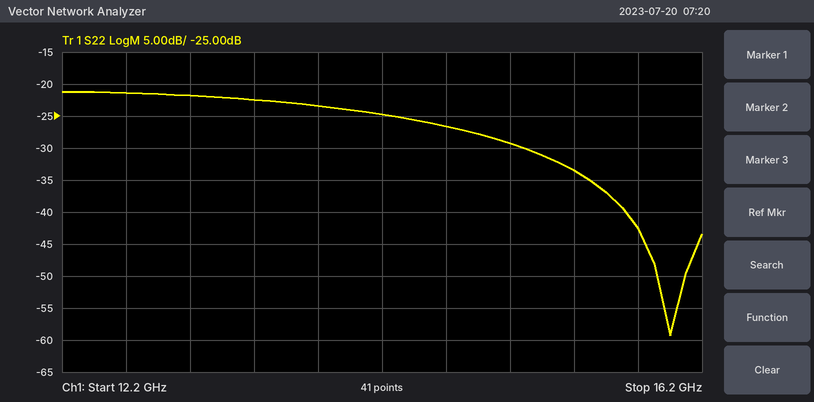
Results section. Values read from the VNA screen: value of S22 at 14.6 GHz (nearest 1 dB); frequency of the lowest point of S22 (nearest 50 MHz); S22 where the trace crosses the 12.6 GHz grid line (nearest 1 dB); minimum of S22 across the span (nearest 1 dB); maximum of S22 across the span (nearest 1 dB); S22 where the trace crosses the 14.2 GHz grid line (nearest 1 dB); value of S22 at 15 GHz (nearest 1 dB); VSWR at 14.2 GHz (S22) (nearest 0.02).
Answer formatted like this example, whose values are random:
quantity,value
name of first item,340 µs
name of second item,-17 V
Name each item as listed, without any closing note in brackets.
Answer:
quantity,value
value of S22 at 14.6 GHz,-27 dB
frequency of the lowest point of S22,16.00 GHz
S22 where the trace crosses the 12.6 GHz grid line,-21 dB
minimum of S22 across the span,-59 dB
maximum of S22 across the span,-21 dB
S22 where the trace crosses the 14.2 GHz grid line,-25 dB
value of S22 at 15 GHz,-29 dB
VSWR at 14.2 GHz (S22),1.12
